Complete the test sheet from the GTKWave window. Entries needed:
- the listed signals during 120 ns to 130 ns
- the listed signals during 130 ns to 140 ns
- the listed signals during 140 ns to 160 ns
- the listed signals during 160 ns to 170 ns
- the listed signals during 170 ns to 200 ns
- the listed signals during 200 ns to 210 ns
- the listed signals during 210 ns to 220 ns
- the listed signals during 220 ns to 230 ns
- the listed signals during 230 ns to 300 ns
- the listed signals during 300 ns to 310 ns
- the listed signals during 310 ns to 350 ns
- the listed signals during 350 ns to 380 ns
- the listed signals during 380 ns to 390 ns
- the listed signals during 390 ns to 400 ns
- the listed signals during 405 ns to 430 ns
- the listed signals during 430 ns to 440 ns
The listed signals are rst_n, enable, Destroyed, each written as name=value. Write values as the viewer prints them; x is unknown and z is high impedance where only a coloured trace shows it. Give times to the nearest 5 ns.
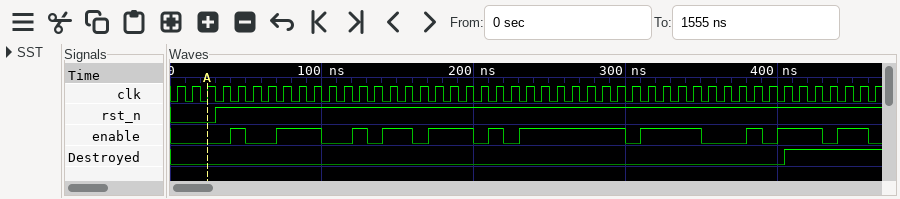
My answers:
rst_n=1, enable=1, Destroyed=0
rst_n=1, enable=0, Destroyed=0
rst_n=1, enable=1, Destroyed=0
rst_n=1, enable=0, Destroyed=0
rst_n=1, enable=1, Destroyed=0
rst_n=1, enable=0, Destroyed=0
rst_n=1, enable=1, Destroyed=0
rst_n=1, enable=0, Destroyed=0
rst_n=1, enable=1, Destroyed=0
rst_n=1, enable=0, Destroyed=0
rst_n=1, enable=1, Destroyed=0
rst_n=1, enable=0, Destroyed=0
rst_n=1, enable=1, Destroyed=0
rst_n=1, enable=0, Destroyed=0
rst_n=1, enable=1, Destroyed=1
rst_n=1, enable=0, Destroyed=1
